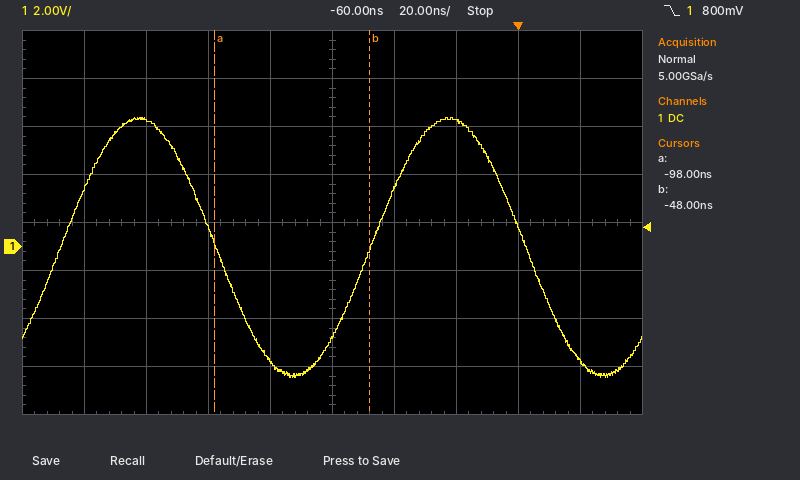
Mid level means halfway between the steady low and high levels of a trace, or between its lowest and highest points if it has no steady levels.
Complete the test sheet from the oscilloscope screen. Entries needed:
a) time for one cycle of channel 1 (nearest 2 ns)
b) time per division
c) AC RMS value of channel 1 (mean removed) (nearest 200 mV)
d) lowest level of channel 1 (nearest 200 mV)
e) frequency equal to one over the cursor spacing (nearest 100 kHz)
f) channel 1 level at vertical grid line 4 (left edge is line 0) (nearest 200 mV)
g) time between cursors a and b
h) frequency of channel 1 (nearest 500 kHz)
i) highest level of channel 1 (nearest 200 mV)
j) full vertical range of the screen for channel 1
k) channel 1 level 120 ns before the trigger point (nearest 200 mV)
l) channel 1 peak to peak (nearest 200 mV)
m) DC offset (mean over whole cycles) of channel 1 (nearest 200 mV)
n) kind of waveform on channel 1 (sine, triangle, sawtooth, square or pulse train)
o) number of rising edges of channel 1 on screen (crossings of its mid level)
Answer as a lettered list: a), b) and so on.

a) 100 ns
b) 20 ns
c) 3.8 V
d) -5.4 V
e) 20.0 MHz
f) -4.8 V
g) 50 ns
h) 10.0 MHz
i) 5.4 V
j) 16 V
k) 5.2 V
l) 10.8 V
m) 0.0 V
n) sine
o) 2
